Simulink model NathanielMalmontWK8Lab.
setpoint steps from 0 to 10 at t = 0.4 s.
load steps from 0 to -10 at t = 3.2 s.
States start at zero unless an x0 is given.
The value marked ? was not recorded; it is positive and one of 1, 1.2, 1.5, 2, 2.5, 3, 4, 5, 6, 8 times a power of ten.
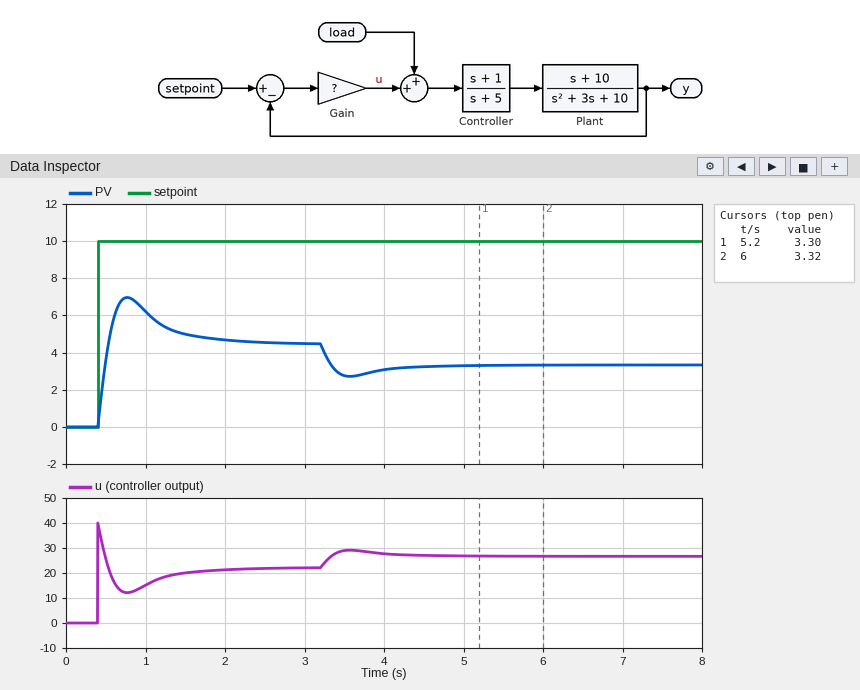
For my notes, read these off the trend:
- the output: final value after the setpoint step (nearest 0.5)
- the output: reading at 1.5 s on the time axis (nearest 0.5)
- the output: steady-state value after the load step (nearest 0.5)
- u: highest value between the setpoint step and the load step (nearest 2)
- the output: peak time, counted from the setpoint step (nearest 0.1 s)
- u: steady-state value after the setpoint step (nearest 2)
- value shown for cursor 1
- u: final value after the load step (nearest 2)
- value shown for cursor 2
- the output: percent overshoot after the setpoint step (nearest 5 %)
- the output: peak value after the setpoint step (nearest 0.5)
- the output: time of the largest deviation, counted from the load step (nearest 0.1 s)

4.5
5.0
3.5
40
0.4 s
22
3.30
26
3.32
55 %
7.0
0.4 s
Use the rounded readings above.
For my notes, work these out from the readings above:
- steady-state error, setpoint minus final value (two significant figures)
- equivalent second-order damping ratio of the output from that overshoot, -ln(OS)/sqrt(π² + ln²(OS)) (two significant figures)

5.5
0.19
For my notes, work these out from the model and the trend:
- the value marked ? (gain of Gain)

4
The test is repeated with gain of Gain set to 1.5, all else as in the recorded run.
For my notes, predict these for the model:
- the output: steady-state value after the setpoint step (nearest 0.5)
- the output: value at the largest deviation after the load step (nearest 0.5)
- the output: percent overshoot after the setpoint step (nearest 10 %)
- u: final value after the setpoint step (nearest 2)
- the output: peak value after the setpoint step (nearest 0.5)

2.5
-0.5
80 %
12
4.0
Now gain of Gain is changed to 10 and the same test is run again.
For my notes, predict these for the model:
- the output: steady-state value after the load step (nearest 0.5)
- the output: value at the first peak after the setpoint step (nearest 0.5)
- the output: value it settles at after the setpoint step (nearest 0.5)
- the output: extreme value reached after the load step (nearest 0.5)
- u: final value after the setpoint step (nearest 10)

6.0
9.0
6.5
6.0
30
